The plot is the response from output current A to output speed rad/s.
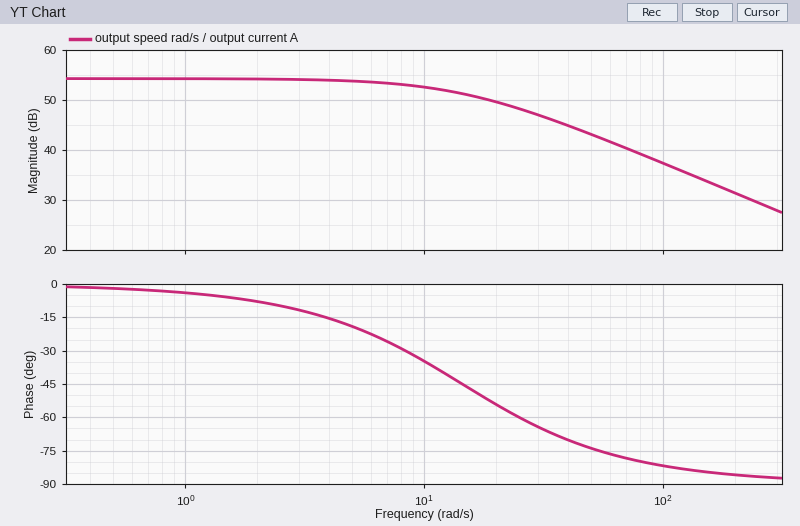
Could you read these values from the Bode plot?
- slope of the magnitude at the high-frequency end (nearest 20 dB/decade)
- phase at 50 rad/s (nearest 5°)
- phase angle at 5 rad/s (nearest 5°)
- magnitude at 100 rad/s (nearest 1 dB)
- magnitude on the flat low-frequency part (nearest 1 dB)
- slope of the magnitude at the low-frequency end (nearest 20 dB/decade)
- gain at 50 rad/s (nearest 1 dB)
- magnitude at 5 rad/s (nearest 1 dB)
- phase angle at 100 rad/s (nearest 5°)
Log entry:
-20 dB/decade
-75°
-20°
37 dB
54 dB
0 dB/decade
43 dB
54 dB
-80°
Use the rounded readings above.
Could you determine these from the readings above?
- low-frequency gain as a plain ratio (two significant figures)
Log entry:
500
